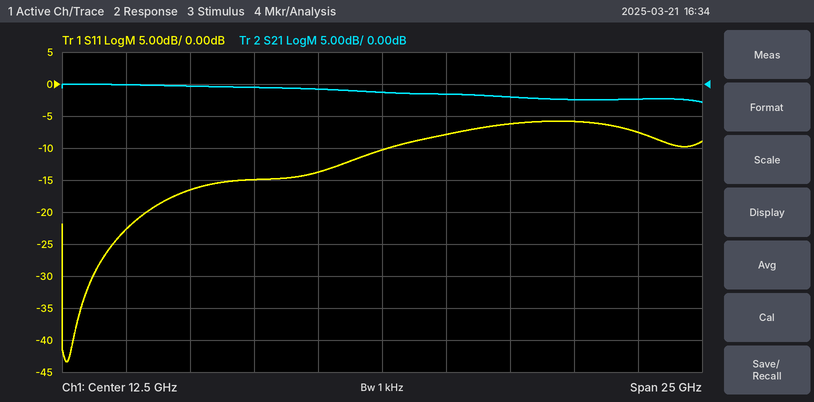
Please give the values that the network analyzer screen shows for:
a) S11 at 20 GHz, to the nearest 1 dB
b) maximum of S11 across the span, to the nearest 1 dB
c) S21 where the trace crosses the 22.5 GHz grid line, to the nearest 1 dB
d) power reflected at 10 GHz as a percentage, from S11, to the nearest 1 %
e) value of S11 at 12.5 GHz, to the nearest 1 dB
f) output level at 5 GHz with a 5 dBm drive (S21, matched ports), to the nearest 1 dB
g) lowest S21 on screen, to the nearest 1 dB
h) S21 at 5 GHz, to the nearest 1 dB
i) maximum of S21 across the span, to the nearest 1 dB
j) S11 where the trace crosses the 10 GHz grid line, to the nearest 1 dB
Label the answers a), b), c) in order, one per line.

a) -6 dB
b) -6 dB
c) -2 dB
d) 4 %
e) -10 dB
f) 5 dBm
g) -3 dB
h) 0 dB
i) 0 dB
j) -14 dB
